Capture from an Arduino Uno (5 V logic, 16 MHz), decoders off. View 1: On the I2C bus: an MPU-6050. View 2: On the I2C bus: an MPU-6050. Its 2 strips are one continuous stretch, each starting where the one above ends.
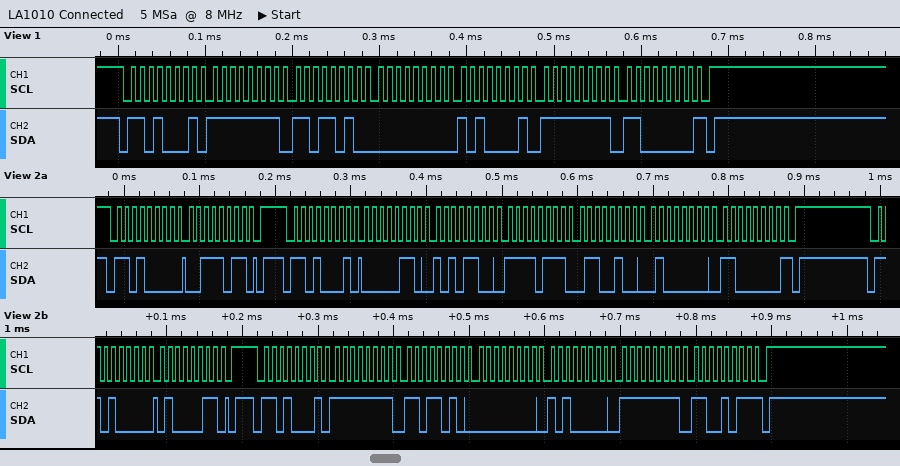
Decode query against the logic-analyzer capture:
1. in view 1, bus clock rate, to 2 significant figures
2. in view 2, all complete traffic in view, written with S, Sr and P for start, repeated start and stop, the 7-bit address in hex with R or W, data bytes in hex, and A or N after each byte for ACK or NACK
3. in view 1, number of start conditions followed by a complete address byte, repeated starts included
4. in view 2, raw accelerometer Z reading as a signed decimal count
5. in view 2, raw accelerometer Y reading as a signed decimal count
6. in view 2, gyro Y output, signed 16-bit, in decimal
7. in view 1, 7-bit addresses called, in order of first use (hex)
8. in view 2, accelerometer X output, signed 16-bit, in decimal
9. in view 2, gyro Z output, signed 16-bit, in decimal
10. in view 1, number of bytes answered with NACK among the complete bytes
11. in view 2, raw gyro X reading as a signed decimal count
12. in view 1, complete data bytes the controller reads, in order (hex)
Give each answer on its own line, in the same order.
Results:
100 kHz
S 68W A 3B A P S 68R A 06 A AC A F7 A 64 A 40 A C0 N P S 68W A 43 A P S 68R A FF A DA A 00 A A0 A FF A CB N P
1
16576
-2204
160
0x68
1708
-53
1
-38
FF DA 00 A1 FF C0
